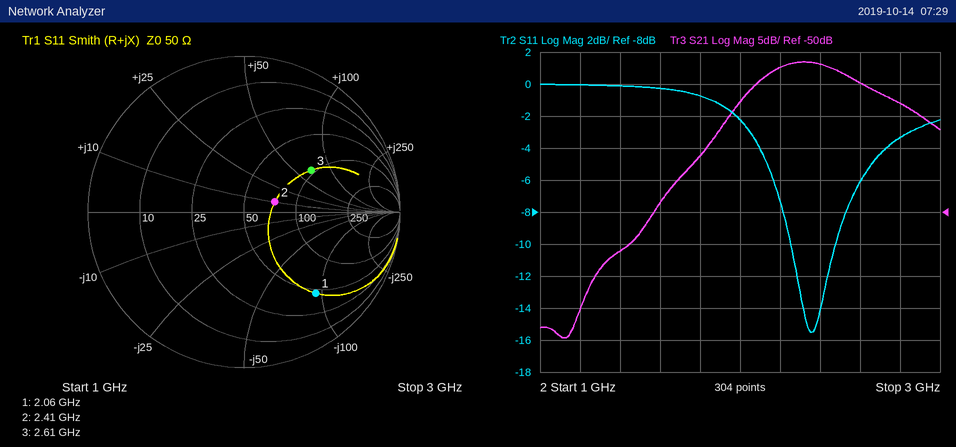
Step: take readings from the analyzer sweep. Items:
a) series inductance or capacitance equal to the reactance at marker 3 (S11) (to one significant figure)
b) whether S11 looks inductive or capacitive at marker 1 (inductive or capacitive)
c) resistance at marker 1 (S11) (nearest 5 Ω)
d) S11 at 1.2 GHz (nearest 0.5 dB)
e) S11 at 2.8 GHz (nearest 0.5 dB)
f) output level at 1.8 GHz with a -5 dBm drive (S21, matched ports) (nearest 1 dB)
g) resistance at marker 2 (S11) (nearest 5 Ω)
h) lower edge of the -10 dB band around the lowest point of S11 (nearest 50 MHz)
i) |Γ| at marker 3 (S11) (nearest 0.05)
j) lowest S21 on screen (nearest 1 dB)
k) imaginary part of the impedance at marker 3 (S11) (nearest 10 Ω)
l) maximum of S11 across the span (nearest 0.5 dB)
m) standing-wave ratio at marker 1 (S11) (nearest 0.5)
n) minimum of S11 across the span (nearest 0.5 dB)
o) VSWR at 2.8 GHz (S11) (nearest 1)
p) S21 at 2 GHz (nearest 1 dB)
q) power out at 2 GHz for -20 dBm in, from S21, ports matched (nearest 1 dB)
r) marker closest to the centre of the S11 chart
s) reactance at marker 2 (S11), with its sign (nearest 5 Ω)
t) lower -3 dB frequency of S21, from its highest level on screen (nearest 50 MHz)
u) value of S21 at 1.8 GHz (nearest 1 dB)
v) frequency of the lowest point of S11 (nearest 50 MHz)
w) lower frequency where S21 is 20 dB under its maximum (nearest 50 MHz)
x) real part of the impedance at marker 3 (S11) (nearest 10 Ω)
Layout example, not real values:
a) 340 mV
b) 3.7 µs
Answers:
a) 4 nH
b) capacitive
c) 45 Ω
d) 0.0 dB
e) -3.5 dB
f) -46 dBm
g) 75 Ω
h) 2.25 GHz
i) 0.50
j) -70 dB
k) +70 Ω
l) 0.0 dB
m) 5.5
n) -15.5 dB
o) 5
p) -33 dB
q) -53 dBm
r) marker 2
s) +10 Ω
t) 2.10 GHz
u) -41 dB
v) 2.35 GHz
w) 1.65 GHz
x) 90 Ω
